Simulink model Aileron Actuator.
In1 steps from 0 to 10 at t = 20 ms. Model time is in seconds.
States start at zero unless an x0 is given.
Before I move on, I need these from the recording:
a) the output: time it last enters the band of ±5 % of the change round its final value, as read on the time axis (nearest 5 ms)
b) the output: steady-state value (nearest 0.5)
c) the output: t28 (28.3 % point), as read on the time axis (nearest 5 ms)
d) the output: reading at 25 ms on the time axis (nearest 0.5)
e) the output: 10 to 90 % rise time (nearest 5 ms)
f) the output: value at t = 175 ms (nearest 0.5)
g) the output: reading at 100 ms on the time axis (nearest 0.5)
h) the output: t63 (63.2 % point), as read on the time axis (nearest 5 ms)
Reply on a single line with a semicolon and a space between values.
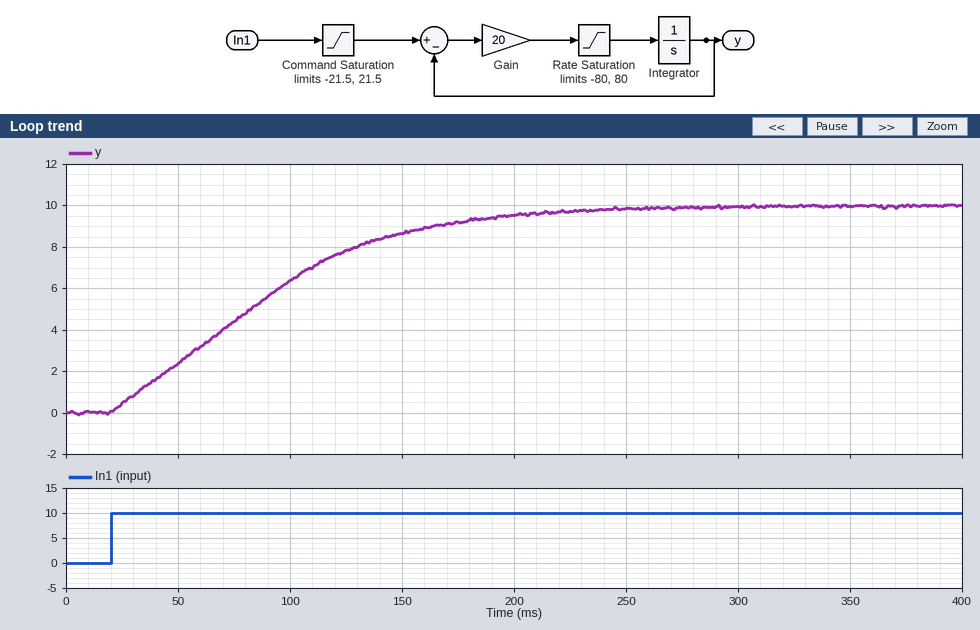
200 ms; 10.0; 55 ms; 0.5; 130 ms; 9.0; 6.5; 100 ms
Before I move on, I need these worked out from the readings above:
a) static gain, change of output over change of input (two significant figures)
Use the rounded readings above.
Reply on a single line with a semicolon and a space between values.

1.0
